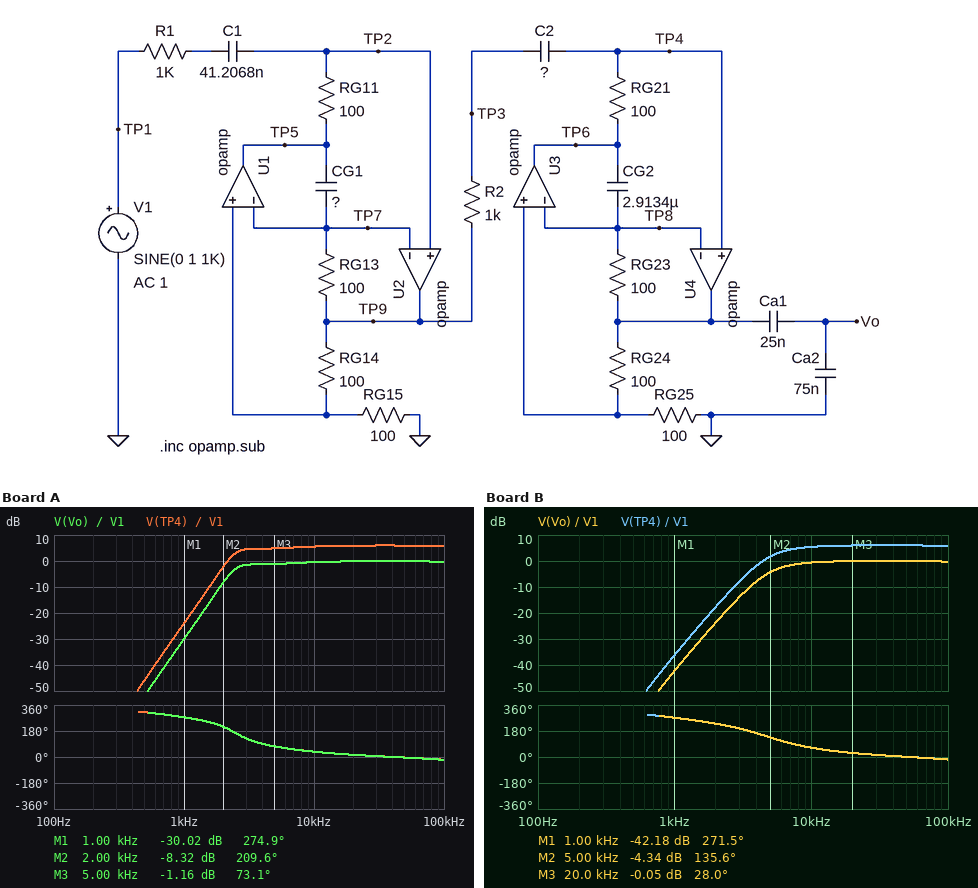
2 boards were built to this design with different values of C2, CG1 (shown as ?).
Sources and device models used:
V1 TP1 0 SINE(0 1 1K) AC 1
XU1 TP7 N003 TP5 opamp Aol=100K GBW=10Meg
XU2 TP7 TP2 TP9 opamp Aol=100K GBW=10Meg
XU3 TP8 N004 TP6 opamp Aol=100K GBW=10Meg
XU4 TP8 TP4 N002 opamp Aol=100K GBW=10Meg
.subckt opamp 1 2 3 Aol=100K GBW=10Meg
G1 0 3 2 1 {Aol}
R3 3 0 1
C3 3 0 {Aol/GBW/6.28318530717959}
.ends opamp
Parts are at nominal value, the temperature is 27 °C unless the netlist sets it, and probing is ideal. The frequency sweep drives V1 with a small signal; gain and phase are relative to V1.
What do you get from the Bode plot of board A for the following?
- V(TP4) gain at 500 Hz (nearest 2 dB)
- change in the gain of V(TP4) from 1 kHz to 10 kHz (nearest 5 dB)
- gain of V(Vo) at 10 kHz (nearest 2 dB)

-46 dB
30 dB
0 dB
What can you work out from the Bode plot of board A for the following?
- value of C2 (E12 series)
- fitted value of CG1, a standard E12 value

270 nF
10 µF
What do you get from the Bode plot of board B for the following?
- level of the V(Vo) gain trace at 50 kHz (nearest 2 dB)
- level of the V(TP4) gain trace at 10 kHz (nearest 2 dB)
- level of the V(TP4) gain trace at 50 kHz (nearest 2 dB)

0 dB
6 dB
6 dB
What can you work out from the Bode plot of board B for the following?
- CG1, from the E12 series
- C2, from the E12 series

2.7 µF
330 nF
